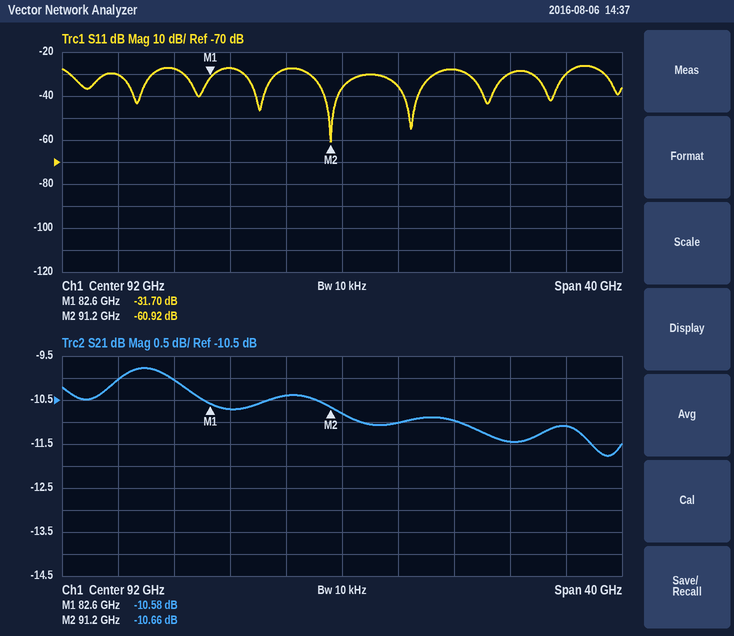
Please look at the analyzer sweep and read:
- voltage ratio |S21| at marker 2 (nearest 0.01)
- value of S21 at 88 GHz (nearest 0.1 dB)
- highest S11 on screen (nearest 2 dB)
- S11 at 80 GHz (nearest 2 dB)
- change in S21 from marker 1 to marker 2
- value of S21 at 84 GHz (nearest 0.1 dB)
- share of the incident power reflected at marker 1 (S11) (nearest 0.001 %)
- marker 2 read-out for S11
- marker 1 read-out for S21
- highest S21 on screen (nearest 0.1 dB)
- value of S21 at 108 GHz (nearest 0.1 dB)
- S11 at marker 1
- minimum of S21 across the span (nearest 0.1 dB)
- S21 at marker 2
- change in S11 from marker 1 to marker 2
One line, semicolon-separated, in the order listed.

0.29; -10.4 dB; -26 dB; -28 dB; -0.08 dB; -10.7 dB; 0.068 %; -60.92 dB; -10.58 dB; -9.8 dB; -11.1 dB; -31.70 dB; -11.8 dB; -10.66 dB; -29.22 dB
